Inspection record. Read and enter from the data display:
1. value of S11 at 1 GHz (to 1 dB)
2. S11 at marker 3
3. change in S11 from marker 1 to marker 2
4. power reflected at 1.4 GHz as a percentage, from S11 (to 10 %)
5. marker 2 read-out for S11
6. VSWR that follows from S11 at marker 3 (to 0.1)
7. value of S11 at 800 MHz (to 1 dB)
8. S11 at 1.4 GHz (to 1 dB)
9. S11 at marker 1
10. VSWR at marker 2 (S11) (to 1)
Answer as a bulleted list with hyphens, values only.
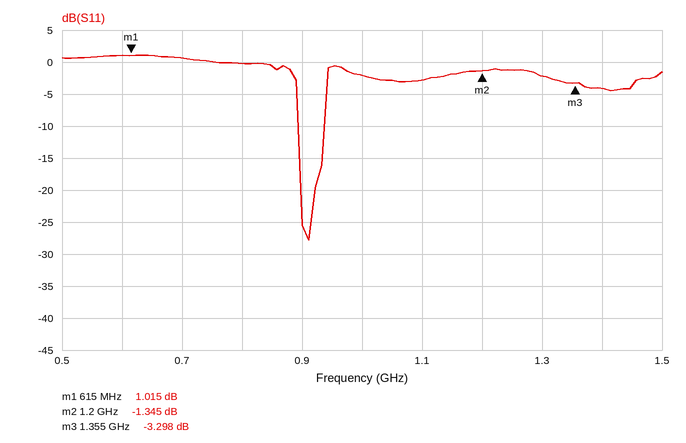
- -2 dB
- -3.298 dB
- -2.360 dB
- 40 %
- -1.345 dB
- 5.3
- 0 dB
- -4 dB
- 1.015 dB
- 13
